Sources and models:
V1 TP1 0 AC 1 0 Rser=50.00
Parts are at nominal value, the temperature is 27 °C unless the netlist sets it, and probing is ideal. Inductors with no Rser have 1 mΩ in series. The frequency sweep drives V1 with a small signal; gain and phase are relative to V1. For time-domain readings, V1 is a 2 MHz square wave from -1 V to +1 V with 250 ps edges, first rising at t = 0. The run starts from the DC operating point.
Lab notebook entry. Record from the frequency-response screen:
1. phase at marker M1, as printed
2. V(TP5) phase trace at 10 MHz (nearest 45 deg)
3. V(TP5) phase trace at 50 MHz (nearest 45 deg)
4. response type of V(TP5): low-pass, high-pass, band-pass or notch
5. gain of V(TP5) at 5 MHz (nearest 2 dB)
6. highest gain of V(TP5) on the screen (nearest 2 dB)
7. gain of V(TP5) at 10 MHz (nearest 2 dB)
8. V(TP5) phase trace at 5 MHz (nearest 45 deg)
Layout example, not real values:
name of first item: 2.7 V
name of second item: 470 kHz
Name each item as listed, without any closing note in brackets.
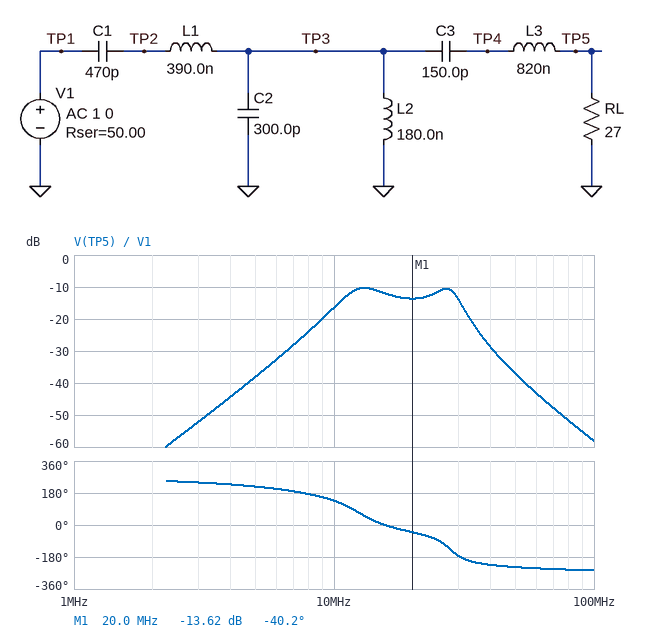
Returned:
phase at marker M1, as printed: -40.2 deg
V(TP5) phase trace at 10 MHz: 135 deg
V(TP5) phase trace at 50 MHz: -225 deg
response type of V(TP5): low-pass, high-pass, band-pass or notch: band-pass
gain of V(TP5) at 5 MHz: -38 dB
highest gain of V(TP5) on the screen: -10 dB
gain of V(TP5) at 10 MHz: -16 dB
V(TP5) phase trace at 5 MHz: 225 deg
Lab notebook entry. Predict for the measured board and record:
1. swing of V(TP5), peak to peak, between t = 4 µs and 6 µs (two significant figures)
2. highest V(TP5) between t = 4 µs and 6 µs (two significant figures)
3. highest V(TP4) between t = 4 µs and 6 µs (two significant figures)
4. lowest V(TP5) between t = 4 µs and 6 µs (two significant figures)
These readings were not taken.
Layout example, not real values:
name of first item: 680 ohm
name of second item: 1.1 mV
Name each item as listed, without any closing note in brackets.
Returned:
swing of V(TP5), peak to peak, between t = 4 µs and 6 µs: 390 mV
highest V(TP5) between t = 4 µs and 6 µs: 190 mV
highest V(TP4) between t = 4 µs and 6 µs: 730 mV
lowest V(TP5) between t = 4 µs and 6 µs: -190 mV
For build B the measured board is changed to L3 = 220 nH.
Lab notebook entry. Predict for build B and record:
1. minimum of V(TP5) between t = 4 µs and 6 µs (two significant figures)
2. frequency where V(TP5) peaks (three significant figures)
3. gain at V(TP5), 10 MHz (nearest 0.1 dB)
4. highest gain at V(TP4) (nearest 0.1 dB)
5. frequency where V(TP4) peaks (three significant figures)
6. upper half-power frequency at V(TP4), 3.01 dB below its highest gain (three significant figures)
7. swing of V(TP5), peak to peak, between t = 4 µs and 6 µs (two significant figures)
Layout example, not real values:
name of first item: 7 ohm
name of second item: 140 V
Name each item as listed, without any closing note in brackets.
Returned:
minimum of V(TP5) between t = 4 µs and 6 µs: -240 mV
frequency where V(TP5) peaks: 18.9 MHz
gain at V(TP5), 10 MHz: -20.8 dB
highest gain at V(TP4): -5.4 dB
frequency where V(TP4) peaks: 34.5 MHz
upper half-power frequency at V(TP4), 3.01 dB below its highest gain: 41.9 MHz
swing of V(TP5), peak to peak, between t = 4 µs and 6 µs: 480 mV
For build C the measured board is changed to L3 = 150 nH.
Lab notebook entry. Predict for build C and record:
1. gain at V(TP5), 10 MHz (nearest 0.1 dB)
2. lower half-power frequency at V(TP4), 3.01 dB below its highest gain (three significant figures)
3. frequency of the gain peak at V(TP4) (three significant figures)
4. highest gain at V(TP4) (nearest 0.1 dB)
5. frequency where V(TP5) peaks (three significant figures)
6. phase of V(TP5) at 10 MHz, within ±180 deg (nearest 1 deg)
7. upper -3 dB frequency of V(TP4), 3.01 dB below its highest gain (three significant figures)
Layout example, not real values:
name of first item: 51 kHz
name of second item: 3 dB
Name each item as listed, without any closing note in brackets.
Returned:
gain at V(TP5), 10 MHz: -21.2 dB
lower half-power frequency at V(TP4), 3.01 dB below its highest gain: 15.7 MHz
frequency of the gain peak at V(TP4): 20.2 MHz
highest gain at V(TP4): -7.0 dB
frequency where V(TP5) peaks: 19.6 MHz
phase of V(TP5) at 10 MHz, within ±180 deg: 154 deg
upper -3 dB frequency of V(TP4), 3.01 dB below its highest gain: 40.7 MHz
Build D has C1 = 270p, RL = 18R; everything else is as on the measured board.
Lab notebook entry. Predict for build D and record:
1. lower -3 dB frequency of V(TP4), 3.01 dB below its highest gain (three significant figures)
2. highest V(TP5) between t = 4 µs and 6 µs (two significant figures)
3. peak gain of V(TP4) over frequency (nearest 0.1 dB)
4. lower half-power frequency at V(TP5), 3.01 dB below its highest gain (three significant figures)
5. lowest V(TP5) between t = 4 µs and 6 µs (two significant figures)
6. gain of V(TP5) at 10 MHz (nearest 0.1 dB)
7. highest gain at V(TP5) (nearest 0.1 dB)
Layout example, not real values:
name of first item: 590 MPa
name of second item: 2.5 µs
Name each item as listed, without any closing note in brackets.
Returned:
lower -3 dB frequency of V(TP4), 3.01 dB below its highest gain: 23.3 MHz
highest V(TP5) between t = 4 µs and 6 µs: 140 mV
peak gain of V(TP4) over frequency: 4.1 dB
lower half-power frequency at V(TP5), 3.01 dB below its highest gain: 11.2 MHz
lowest V(TP5) between t = 4 µs and 6 µs: -140 mV
gain of V(TP5) at 10 MHz: -19.3 dB
highest gain at V(TP5): -10.9 dB
